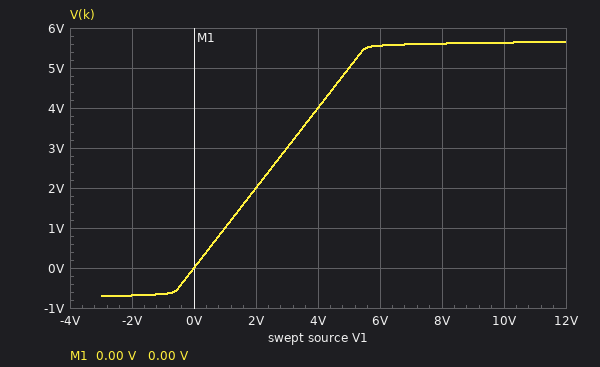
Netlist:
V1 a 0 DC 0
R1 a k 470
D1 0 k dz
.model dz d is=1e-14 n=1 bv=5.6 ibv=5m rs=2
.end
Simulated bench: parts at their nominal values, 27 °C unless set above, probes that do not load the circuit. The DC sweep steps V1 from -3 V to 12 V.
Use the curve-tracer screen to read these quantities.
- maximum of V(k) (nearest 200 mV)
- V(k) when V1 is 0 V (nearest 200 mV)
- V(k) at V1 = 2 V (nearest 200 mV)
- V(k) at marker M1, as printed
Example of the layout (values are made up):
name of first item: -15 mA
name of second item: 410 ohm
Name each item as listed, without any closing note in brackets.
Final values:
maximum of V(k): 5.6 V
V(k) when V1 is 0 V: 0 V
V(k) at V1 = 2 V: 2.0 V
V(k) at marker M1, as printed: 0.00 V
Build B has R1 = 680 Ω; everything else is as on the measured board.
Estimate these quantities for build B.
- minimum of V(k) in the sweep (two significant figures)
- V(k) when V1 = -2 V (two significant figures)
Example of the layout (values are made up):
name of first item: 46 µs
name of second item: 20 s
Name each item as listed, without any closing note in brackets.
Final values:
minimum of V(k) in the sweep: -690 mV
V(k) when V1 = -2 V: -680 mV
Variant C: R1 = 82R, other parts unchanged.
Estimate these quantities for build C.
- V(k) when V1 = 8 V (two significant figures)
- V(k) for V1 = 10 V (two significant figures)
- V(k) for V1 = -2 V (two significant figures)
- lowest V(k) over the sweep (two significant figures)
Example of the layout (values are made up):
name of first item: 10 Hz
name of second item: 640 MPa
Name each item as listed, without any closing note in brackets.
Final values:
V(k) when V1 = 8 V: 5.7 V
V(k) for V1 = 10 V: 5.8 V
V(k) for V1 = -2 V: -760 mV
lowest V(k) over the sweep: -790 mV
